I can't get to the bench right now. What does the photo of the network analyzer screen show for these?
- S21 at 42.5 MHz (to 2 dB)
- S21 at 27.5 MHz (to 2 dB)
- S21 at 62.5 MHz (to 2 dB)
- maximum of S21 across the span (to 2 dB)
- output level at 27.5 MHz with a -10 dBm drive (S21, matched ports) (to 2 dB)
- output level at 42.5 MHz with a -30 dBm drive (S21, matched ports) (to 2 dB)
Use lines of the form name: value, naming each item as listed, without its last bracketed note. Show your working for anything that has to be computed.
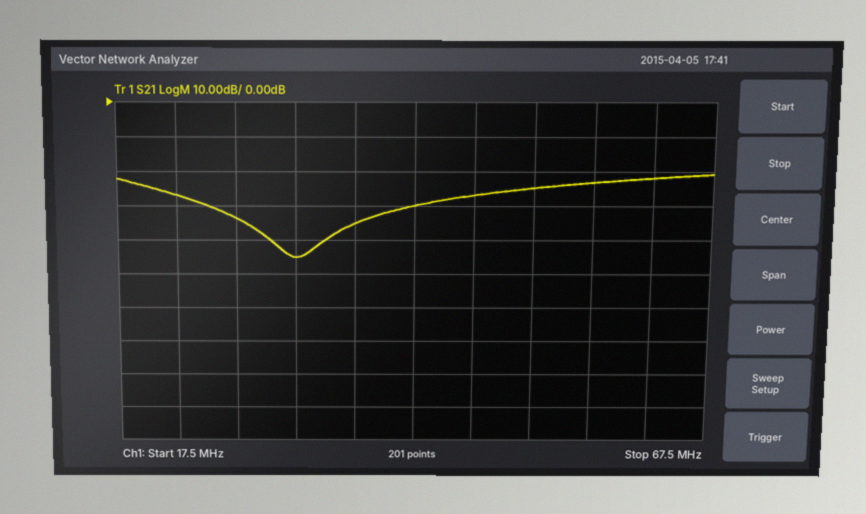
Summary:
S21 at 42.5 MHz: -30 dB
S21 at 27.5 MHz: -34 dB
S21 at 62.5 MHz: -22 dB
maximum of S21 across the span: -20 dB
output level at 27.5 MHz with a -10 dBm drive (S21, matched ports): -10 dBm + (-34 dB) = -44 dBm
output level at 42.5 MHz with a -30 dBm drive (S21, matched ports): -30 dBm + (-30 dB) = -60 dBm
